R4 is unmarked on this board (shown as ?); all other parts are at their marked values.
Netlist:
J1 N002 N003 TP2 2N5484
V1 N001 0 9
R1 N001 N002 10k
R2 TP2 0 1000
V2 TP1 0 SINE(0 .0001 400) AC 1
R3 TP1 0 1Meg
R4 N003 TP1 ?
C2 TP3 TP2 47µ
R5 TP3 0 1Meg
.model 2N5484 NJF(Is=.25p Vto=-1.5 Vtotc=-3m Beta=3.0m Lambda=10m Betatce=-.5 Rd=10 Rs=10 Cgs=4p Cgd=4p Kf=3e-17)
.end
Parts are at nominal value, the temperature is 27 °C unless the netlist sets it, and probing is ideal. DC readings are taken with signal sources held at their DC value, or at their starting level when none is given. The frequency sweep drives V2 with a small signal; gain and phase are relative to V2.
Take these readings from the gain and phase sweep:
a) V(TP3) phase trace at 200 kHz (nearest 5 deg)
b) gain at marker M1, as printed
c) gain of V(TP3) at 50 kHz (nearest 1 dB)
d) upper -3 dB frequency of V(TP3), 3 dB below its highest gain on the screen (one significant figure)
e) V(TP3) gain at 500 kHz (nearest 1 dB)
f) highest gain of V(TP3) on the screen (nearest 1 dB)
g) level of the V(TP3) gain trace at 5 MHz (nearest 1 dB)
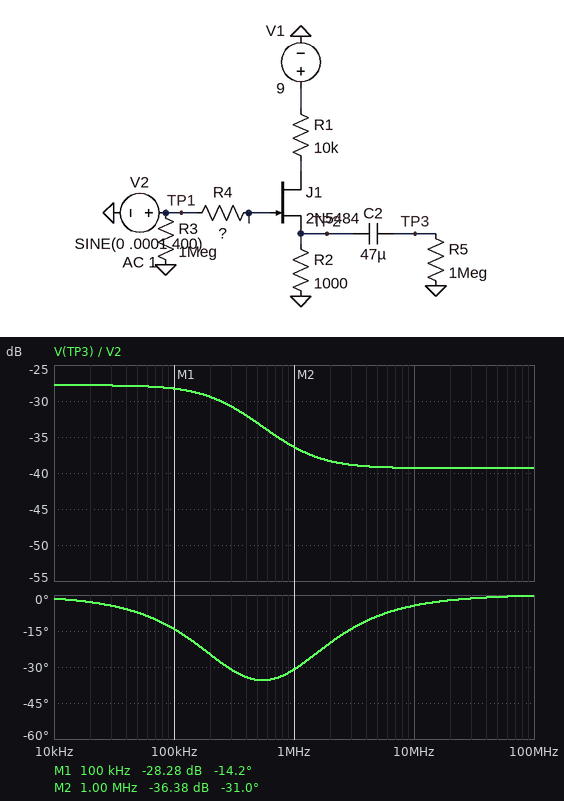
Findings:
-25 deg
-28.28 dB
-28 dB
300 kHz
-33 dB
-28 dB
-39 dB
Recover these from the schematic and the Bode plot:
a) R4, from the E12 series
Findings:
82 kΩ
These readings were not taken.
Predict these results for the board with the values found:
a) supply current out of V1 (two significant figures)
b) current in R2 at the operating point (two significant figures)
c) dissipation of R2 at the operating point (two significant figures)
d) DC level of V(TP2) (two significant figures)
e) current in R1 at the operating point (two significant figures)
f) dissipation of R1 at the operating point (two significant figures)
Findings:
800 µA
800 µA
630 µW
800 mV
800 µA
6.3 mW
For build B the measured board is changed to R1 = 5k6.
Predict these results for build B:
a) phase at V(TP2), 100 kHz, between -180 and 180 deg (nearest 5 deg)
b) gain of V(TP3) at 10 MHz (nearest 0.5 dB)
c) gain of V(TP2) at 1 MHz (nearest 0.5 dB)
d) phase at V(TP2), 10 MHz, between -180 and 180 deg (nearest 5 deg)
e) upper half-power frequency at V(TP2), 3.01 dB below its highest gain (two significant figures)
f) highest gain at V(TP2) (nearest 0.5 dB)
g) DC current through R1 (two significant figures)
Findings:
-30 deg
-35.5 dB
-17.0 dB
-55 deg
190 kHz
-2.5 dB
940 µA
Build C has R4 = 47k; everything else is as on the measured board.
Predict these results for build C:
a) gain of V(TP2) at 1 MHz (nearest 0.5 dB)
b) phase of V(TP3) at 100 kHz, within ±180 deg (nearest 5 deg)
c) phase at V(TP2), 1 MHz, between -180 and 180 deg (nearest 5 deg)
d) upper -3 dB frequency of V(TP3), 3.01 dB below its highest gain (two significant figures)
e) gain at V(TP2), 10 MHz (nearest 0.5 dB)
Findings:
-32.0 dB
-5 deg
-20 deg
640 kHz
-34.5 dB
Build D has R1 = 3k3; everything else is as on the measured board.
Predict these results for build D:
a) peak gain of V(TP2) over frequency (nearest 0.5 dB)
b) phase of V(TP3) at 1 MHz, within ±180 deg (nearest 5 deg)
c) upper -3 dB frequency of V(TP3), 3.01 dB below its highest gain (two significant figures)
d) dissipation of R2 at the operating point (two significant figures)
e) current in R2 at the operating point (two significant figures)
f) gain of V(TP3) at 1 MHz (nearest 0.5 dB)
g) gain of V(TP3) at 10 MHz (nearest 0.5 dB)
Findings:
-2.5 dB
-70 deg
320 kHz
890 µW
940 µA
-12.5 dB
-32.0 dB
